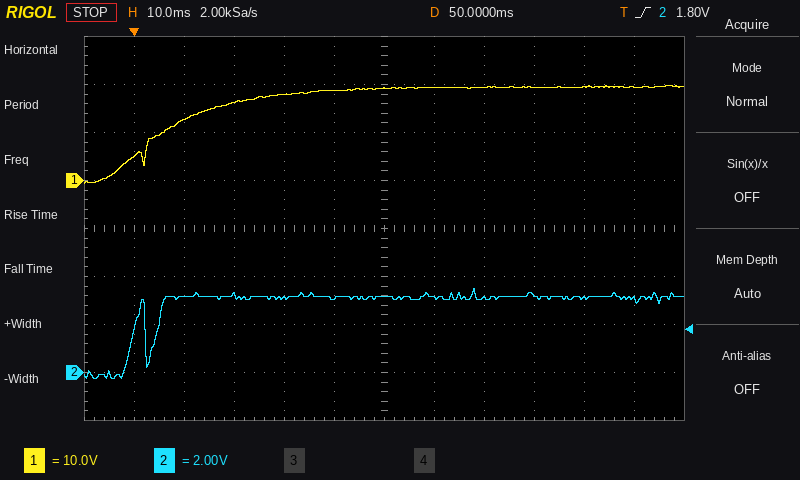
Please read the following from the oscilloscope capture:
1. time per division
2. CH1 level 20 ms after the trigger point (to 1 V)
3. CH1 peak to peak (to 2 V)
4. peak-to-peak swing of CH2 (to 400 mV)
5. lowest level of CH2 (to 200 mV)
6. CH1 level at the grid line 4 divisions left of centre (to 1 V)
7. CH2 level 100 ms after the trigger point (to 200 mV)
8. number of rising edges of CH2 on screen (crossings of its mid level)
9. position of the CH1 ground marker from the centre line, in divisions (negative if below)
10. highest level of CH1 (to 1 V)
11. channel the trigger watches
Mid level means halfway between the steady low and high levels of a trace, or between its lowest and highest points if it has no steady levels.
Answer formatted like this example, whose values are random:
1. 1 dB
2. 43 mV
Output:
1. 10 ms
2. 16 V
3. 20 V
4. 3.6 V
5. -200 mV
6. 13 V
7. 3.0 V
8. 2
9. +1.0 div
10. 20 V
11. CH2
